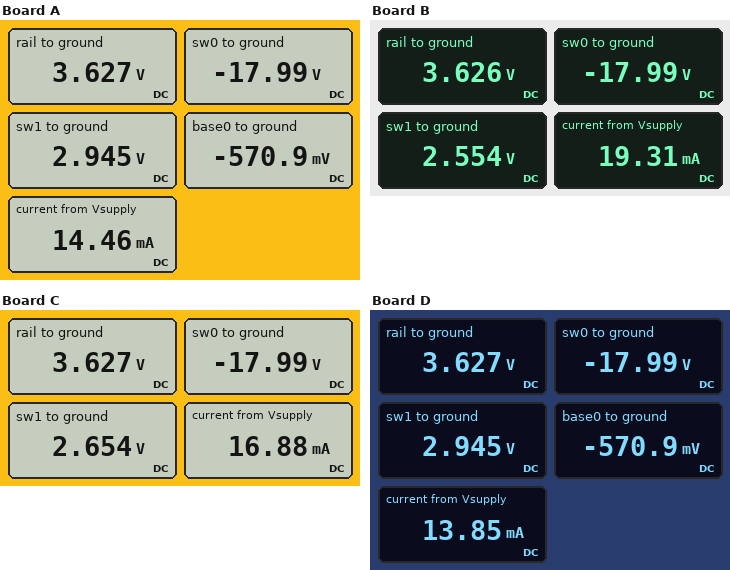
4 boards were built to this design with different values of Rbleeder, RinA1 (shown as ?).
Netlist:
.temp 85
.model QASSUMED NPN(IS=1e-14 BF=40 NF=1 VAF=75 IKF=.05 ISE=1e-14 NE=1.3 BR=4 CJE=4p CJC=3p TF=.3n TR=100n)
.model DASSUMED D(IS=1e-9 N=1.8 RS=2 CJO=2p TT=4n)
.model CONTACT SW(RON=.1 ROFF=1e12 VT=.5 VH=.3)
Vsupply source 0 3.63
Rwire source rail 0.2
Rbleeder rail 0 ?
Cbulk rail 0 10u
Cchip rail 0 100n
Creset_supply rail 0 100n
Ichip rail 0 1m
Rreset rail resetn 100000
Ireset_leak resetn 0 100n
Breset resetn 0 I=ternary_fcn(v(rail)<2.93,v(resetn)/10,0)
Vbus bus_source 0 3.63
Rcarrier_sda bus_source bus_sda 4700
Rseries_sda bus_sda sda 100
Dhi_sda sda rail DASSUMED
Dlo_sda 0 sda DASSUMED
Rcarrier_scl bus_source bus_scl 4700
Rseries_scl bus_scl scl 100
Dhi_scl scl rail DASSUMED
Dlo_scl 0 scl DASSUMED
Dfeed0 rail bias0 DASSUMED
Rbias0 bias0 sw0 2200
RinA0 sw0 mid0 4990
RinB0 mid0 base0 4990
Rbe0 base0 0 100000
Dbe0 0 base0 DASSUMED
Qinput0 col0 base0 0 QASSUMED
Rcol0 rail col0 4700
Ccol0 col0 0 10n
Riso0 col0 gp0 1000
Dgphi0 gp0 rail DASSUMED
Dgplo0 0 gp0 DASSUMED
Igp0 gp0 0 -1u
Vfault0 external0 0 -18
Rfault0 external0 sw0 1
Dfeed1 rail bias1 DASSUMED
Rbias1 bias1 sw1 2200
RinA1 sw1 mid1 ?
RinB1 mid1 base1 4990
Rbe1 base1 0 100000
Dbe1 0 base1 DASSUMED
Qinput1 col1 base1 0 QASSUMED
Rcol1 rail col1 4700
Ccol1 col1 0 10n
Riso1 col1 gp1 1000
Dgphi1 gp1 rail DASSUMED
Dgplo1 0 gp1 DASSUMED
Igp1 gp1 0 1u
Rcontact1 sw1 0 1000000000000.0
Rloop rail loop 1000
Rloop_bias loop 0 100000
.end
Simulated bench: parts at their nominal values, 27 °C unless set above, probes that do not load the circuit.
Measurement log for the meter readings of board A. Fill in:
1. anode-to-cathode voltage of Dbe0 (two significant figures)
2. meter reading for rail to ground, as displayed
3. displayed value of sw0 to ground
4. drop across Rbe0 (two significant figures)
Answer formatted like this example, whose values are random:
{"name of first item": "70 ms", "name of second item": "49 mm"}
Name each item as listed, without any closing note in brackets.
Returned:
{"anode-to-cathode voltage of Dbe0": "570 mV", "meter reading for rail to ground, as displayed": "3.627 V", "displayed value of sw0 to ground": "-17.99 V", "drop across Rbe0": "570 mV"}
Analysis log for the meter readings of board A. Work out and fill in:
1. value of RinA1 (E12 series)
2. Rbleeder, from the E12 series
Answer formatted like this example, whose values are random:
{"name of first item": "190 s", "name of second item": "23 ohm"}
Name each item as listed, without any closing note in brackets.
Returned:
{"value of RinA1": "15 kΩ", "Rbleeder, from the E12 series": "1.2 kΩ"}
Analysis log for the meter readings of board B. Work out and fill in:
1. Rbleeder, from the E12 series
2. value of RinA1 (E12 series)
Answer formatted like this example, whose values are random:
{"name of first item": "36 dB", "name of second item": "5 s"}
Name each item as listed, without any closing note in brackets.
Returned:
{"Rbleeder, from the E12 series": "470 Ω", "value of RinA1": "2.2 kΩ"}
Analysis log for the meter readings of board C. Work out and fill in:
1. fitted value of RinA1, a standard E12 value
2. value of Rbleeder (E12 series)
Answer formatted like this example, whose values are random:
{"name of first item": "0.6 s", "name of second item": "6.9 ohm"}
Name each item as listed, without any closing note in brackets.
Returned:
{"fitted value of RinA1, a standard E12 value": "3.9 kΩ", "value of Rbleeder": "680 Ω"}
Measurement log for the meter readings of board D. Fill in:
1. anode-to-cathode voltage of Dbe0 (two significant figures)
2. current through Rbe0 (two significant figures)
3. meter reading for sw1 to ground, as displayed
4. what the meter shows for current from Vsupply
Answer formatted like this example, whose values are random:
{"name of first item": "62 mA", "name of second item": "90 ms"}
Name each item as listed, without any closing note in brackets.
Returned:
{"anode-to-cathode voltage of Dbe0": "570 mV", "current through Rbe0": "5.7 µA", "meter reading for sw1 to ground, as displayed": "2.945 V", "what the meter shows for current from Vsupply": "13.85 mA"}
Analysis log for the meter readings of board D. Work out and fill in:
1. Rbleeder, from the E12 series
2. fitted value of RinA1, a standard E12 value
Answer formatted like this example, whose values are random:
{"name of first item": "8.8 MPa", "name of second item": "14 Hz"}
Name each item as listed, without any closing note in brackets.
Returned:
{"Rbleeder, from the E12 series": "1.5 kΩ", "fitted value of RinA1, a standard E12 value": "15 kΩ"}
